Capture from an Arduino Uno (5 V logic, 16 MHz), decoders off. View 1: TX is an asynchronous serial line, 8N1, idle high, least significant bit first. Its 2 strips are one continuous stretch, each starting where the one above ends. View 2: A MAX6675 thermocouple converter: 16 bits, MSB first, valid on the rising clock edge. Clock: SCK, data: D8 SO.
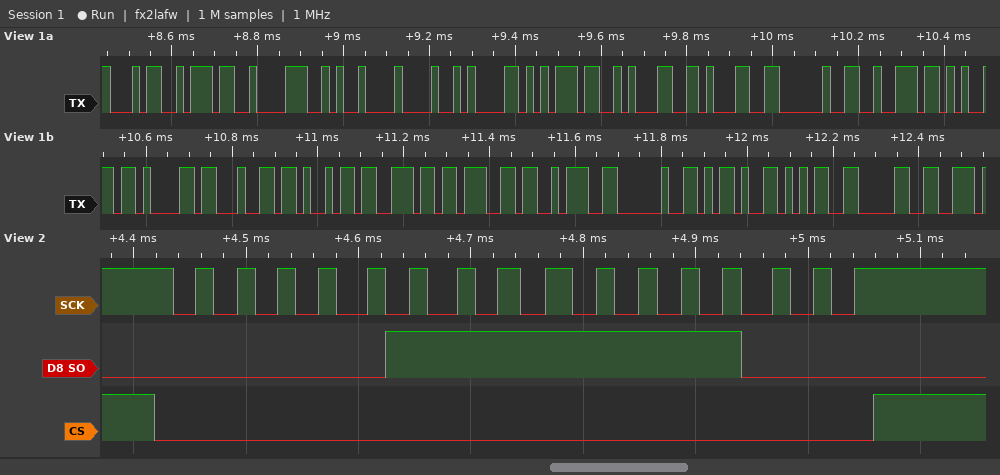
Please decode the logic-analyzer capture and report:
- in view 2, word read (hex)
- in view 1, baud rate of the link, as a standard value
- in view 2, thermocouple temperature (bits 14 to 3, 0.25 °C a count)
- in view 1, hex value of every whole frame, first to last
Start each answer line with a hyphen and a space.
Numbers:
- 0x07F8
- 57600 baud
- 63.75 °C
- 34 37 38 09 48 58 37 31 31 20 72 65 61 64 69 6E 67 3A 20 2D 35 30
